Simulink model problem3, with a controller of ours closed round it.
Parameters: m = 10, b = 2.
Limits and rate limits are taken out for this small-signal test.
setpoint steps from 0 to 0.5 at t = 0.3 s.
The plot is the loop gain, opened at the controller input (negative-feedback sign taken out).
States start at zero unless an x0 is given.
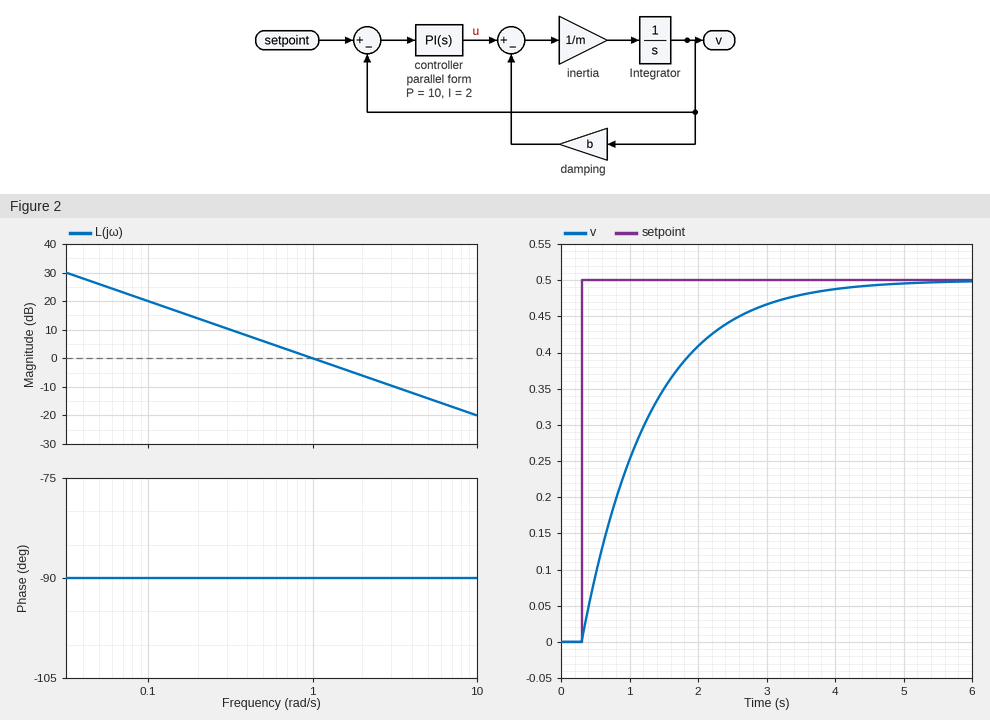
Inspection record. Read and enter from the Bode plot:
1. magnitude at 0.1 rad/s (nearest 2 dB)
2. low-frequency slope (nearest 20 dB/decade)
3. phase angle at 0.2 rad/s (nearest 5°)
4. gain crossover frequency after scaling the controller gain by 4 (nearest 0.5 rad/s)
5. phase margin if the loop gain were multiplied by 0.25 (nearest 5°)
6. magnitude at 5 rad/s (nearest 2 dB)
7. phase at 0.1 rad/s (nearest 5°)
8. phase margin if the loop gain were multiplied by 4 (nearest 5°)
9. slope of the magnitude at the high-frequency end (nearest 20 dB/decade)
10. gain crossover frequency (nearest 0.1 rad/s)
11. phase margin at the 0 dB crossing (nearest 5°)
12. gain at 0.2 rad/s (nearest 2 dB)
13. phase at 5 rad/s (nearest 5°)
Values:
20 dB
-20 dB/decade
-90°
4.0 rad/s
90°
-14 dB
-90°
90°
-20 dB/decade
1.0 rad/s
90°
14 dB
-90°
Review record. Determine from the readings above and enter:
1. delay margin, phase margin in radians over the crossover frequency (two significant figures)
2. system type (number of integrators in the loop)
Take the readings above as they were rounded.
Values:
1.6 s
1
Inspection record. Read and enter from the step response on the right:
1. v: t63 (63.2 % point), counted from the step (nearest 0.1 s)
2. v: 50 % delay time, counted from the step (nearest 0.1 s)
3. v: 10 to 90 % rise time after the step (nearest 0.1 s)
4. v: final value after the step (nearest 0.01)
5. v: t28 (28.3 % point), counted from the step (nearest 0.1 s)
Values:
1.0 s
0.7 s
2.2 s
0.50
0.3 s
